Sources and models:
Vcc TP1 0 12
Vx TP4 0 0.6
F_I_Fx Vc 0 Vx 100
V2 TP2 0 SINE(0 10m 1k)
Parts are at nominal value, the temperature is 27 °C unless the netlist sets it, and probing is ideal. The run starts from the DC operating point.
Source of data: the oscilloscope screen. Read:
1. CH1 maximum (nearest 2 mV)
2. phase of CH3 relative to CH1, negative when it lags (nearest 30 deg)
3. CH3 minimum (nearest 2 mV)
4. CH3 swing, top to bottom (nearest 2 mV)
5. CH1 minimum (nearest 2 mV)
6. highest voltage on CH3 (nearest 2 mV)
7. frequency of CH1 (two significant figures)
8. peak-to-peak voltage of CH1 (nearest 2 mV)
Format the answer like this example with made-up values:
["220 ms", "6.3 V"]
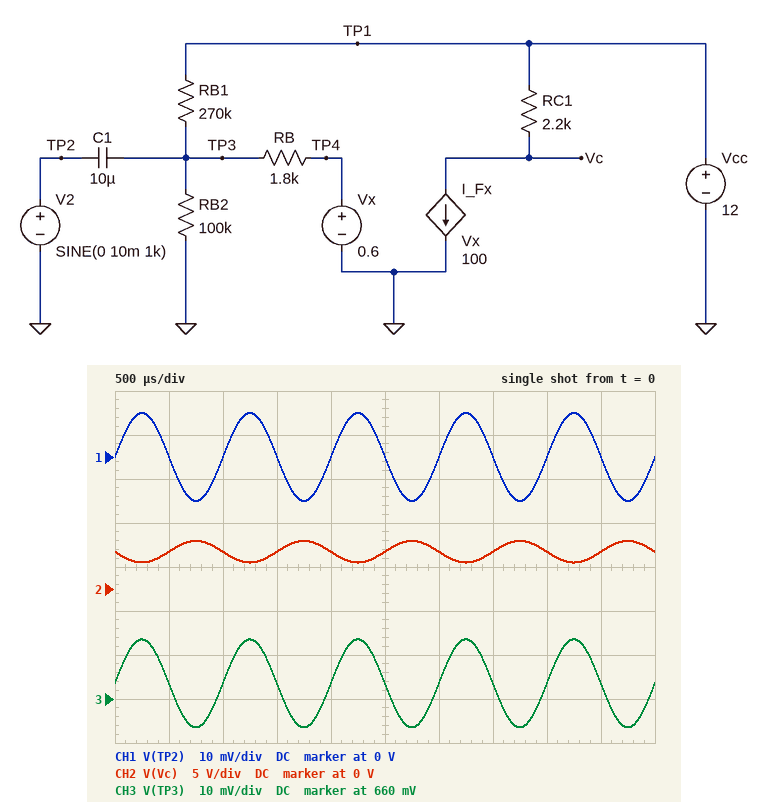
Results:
["10 mV", "0 deg", "654 mV", "20 mV", "-10 mV", "674 mV", "1.0 kHz", "20 mV"]
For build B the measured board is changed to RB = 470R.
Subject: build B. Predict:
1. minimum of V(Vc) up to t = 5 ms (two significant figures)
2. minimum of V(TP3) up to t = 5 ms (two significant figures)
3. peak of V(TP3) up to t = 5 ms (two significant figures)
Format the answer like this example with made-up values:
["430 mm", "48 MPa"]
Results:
["-530 mV", "610 mV", "630 mV"]
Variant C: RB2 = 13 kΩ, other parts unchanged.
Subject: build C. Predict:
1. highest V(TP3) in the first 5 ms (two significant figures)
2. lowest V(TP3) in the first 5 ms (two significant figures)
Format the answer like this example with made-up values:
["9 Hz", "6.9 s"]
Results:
["600 mV", "580 mV"]
